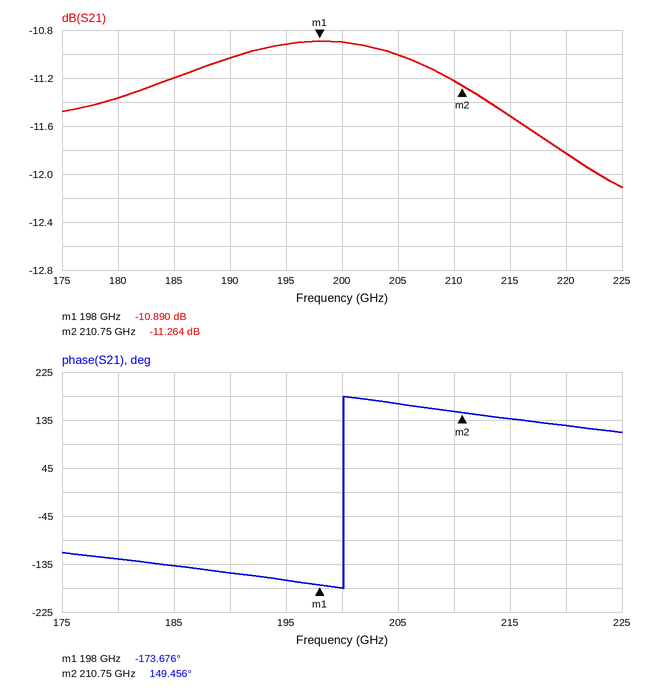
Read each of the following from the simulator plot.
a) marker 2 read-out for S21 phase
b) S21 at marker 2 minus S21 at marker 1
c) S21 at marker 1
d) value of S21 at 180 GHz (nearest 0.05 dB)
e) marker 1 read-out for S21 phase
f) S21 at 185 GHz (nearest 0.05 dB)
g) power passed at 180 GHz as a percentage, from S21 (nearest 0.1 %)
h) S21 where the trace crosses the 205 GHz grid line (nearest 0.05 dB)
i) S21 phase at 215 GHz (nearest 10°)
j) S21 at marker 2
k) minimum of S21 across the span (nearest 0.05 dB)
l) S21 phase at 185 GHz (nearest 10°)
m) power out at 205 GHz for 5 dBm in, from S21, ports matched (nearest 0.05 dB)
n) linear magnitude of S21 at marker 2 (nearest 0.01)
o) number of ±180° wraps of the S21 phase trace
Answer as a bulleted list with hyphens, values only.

- 149.456°
- -0.374 dB
- -10.890 dB
- -11.35 dB
- -173.676°
- -11.20 dB
- 7.3 %
- -11.00 dB
- 140°
- -11.264 dB
- -12.10 dB
- -140°
- -6.00 dBm
- 0.27
- 1
